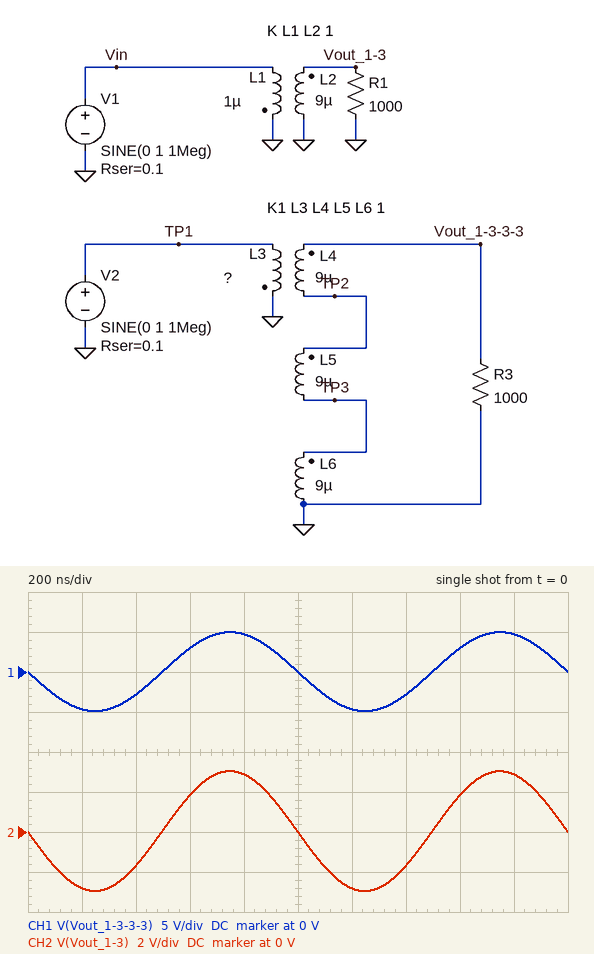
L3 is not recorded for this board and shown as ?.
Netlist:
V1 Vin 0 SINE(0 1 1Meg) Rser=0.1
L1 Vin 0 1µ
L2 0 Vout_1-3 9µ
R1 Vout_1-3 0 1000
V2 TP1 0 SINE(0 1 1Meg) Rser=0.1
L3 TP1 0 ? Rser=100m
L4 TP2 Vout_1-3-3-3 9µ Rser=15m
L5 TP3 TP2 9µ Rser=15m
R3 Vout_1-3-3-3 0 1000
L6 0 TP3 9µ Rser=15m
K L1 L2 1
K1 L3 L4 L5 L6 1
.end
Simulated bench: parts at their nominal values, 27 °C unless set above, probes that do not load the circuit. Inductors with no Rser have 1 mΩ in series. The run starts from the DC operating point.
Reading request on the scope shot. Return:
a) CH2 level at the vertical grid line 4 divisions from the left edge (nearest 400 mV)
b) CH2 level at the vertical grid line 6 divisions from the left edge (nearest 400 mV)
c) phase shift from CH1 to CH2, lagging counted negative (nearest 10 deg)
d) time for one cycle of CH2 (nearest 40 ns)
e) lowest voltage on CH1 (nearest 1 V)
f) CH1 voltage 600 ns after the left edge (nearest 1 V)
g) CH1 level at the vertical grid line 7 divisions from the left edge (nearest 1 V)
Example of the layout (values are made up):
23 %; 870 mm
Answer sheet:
2.8 V; -2.8 V; 0 deg; 1.00 µs; -5 V; 3 V; -3 V
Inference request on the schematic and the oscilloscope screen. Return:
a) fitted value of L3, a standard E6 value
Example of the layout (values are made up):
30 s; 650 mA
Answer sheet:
3.3 µH
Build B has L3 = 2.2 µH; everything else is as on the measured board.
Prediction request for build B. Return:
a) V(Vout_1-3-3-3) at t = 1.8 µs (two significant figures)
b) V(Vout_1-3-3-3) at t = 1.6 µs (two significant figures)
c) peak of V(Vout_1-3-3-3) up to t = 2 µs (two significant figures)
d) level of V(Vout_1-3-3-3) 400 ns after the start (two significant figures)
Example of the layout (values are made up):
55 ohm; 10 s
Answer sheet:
5.8 V; 3.7 V; 6.1 V; -3.4 V
